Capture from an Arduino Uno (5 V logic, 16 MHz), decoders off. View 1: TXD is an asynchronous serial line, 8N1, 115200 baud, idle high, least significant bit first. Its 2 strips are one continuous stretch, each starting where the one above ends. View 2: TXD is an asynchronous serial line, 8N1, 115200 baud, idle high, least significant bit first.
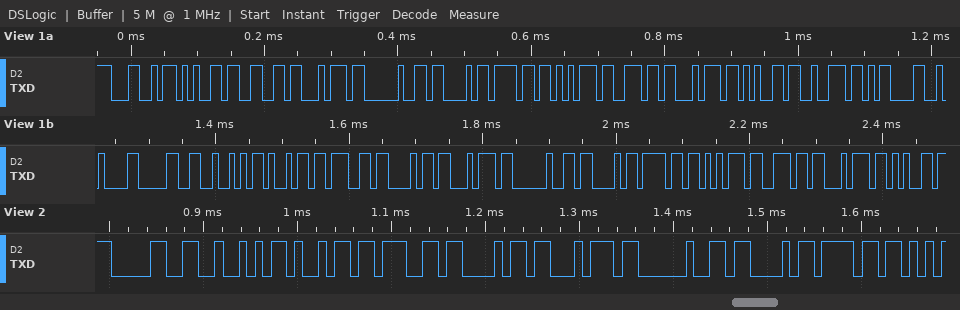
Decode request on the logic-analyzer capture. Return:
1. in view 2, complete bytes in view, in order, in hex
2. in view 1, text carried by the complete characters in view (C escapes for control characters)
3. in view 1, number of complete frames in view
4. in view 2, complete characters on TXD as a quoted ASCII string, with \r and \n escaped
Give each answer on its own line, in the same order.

0x30 0x52 0x69 0x67 0x68 0x74 0x20 0x43 0x6F
"Left Counter\r\n0Right Counte"
27
"0Right Co"
